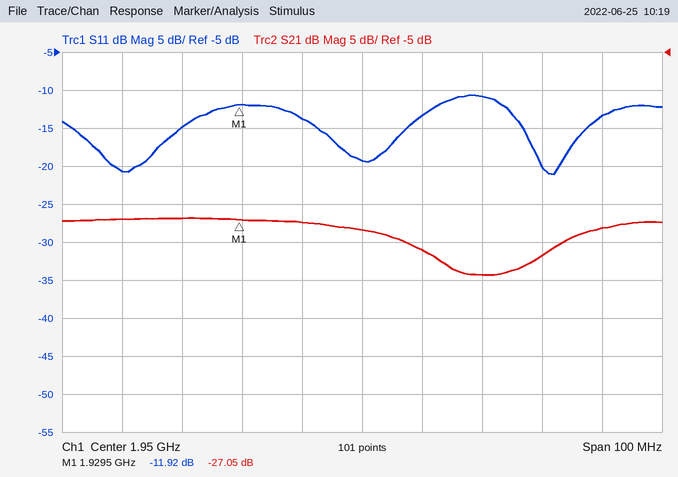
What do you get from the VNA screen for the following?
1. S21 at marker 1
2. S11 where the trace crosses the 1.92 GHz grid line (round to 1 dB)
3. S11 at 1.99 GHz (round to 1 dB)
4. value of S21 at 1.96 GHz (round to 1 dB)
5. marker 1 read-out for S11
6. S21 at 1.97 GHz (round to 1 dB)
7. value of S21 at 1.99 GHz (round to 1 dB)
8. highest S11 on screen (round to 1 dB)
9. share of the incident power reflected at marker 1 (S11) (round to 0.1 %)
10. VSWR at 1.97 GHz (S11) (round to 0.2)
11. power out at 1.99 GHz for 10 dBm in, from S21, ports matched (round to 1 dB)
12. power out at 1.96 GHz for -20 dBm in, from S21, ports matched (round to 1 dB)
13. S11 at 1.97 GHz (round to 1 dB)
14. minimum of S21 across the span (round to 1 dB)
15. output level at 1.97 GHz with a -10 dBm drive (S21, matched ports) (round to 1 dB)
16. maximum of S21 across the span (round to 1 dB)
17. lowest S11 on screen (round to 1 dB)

-27.05 dB
-15 dB
-13 dB
-31 dB
-11.92 dB
-34 dB
-28 dB
-11 dB
6.4 %
1.8
-18 dBm
-51 dBm
-11 dB
-34 dB
-44 dBm
-27 dB
-21 dB
